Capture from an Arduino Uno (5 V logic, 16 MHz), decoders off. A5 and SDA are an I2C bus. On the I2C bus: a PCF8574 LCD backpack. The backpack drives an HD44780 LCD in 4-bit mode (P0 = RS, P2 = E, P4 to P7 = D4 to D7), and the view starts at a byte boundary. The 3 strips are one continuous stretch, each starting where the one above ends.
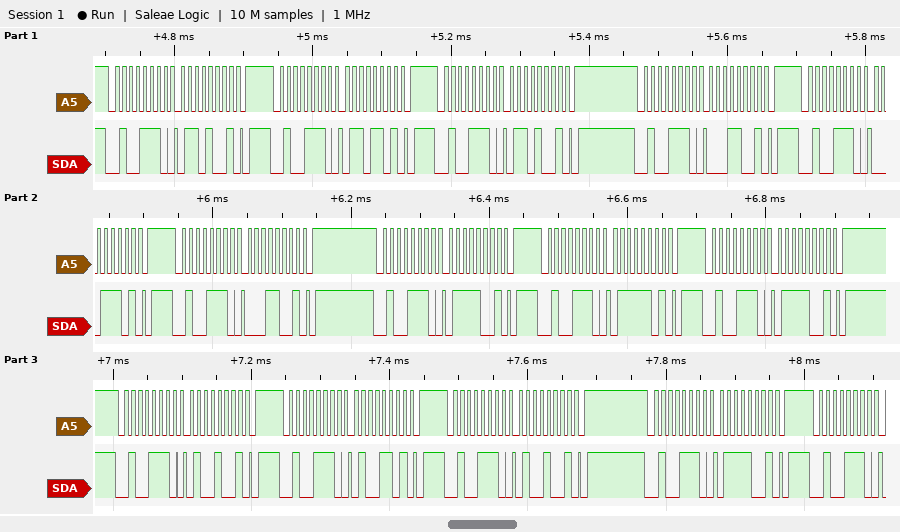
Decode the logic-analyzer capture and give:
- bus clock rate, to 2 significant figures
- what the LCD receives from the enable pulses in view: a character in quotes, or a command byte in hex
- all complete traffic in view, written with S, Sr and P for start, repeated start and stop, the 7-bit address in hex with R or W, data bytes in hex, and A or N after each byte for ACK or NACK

100 kHz
'a' 't'
S 27W A 69 A P S 27W A 6D A P S 27W A 69 A P S 27W A 19 A P S 27W A 1D A P S 27W A 19 A P S 27W A 79 A P S 27W A 7D A P S 27W A 79 A P S 27W A 49 A P S 27W A 4D A P S 27W A 49 A P S 27W A 79 A P S 27W A
